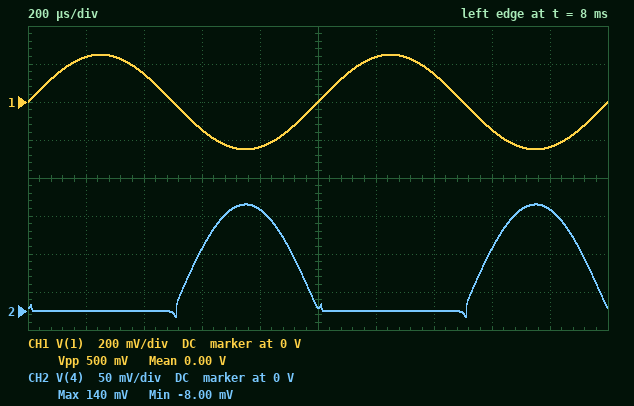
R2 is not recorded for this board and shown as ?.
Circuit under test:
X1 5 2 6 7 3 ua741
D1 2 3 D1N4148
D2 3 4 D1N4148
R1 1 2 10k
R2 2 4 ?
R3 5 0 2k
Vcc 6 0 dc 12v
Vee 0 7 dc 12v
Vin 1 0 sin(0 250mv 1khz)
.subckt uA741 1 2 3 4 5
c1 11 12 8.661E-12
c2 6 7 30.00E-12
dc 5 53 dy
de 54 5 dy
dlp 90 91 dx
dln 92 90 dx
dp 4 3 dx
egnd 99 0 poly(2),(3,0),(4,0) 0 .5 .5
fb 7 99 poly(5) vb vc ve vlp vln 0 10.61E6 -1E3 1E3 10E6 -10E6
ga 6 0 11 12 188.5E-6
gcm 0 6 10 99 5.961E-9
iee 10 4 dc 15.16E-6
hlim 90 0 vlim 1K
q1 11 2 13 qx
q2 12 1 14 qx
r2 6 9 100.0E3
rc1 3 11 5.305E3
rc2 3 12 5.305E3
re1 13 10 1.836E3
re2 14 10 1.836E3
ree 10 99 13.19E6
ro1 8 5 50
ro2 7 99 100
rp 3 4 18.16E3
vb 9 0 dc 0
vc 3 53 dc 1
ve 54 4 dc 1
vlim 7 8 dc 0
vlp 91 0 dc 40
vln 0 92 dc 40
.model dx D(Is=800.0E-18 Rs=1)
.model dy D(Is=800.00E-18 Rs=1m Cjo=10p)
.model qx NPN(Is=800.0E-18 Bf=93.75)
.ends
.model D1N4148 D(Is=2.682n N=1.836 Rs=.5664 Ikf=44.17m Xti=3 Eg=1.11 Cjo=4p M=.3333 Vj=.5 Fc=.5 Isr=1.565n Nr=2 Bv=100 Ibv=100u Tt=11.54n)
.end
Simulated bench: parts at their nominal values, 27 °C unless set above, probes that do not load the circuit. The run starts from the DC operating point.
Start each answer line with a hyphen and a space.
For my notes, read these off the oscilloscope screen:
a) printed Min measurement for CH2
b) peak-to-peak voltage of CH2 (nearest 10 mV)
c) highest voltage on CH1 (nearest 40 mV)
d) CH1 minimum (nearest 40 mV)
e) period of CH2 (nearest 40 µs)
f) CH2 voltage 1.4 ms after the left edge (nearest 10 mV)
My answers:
- -8.00 mV
- 150 mV
- 240 mV
- -240 mV
- 1.00 ms
- 0 V
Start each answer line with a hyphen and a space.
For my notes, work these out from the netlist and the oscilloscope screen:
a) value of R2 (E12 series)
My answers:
- 5.6 kΩ
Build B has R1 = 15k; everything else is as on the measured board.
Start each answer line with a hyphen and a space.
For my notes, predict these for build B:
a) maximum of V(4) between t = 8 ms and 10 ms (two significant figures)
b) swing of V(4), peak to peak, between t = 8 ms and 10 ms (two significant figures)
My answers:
- 94 mV
- 100 mV
